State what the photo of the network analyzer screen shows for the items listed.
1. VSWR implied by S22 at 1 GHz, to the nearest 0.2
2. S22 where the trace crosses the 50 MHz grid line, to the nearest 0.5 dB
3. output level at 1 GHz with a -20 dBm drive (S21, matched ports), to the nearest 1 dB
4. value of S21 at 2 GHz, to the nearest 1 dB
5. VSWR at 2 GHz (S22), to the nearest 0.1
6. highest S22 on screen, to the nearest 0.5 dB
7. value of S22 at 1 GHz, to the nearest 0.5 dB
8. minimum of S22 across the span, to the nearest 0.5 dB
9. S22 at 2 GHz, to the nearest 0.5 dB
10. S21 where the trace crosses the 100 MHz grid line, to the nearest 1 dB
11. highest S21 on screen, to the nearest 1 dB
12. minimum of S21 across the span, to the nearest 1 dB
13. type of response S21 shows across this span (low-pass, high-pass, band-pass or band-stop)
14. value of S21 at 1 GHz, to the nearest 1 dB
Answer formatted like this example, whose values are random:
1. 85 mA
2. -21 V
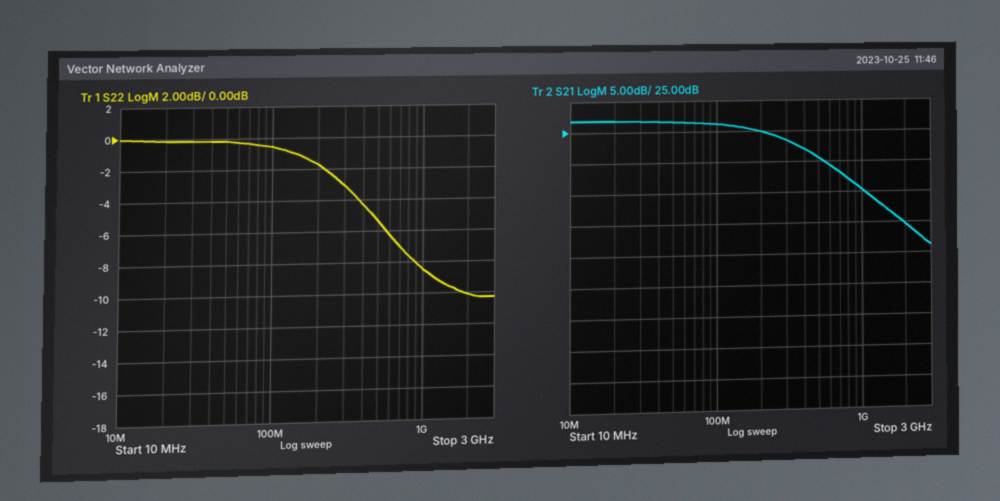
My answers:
1. 2.2
2. 0.0 dB
3. -5 dBm
4. 10 dB
5. 1.9
6. 0.0 dB
7. -8.5 dB
8. -10.5 dB
9. -10.0 dB
10. 26 dB
11. 27 dB
12. 6 dB
13. low-pass
14. 15 dB
